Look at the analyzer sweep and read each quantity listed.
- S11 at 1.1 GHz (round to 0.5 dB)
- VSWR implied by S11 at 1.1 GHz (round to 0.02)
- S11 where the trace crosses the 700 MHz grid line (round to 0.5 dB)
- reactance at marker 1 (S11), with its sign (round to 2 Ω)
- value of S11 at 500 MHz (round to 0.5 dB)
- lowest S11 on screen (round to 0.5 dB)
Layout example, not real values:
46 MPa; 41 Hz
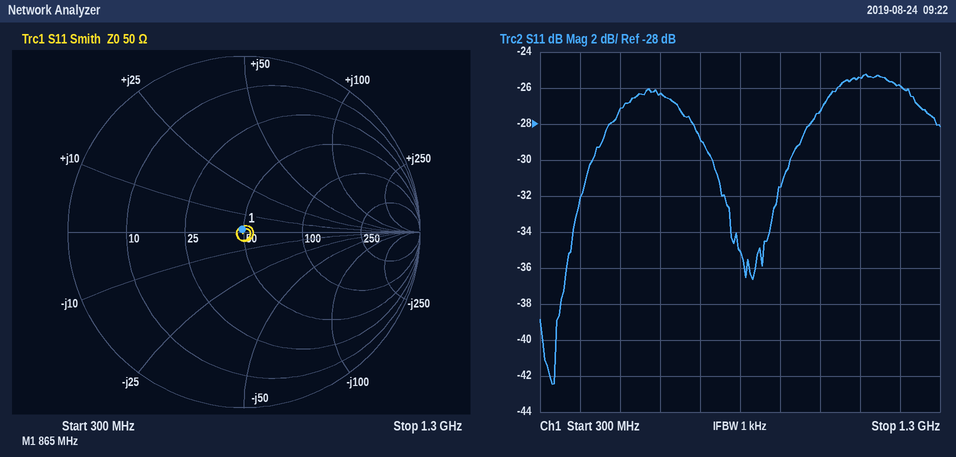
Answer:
-25.5 dB; 1.12; -29.0 dB; +2 Ω; -27.0 dB; -42.5 dB
